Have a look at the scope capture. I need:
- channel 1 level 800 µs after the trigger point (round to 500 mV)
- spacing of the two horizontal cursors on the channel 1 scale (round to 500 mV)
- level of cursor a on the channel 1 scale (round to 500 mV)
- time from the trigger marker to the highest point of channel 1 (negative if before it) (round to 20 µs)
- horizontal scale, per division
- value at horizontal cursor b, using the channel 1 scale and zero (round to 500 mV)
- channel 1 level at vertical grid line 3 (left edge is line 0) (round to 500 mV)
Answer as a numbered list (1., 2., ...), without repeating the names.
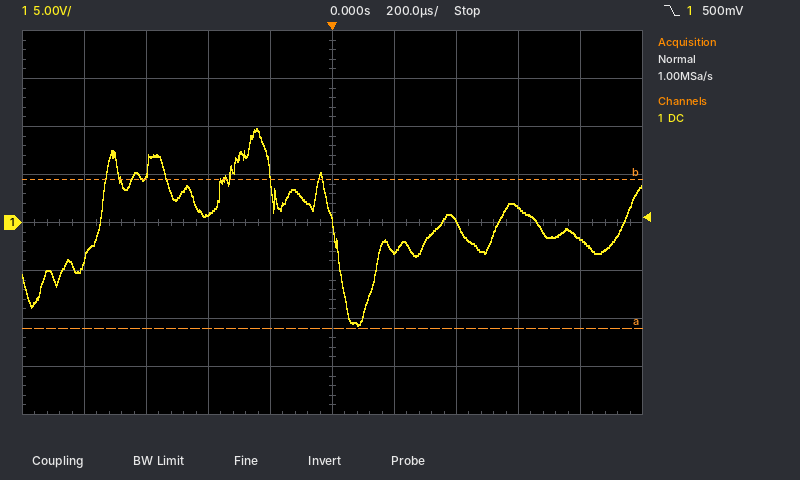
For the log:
1. -2.0 V
2. 15.5 V
3. -11.0 V
4. -240 µs
5. 200 µs
6. 4.5 V
7. 1.0 V
